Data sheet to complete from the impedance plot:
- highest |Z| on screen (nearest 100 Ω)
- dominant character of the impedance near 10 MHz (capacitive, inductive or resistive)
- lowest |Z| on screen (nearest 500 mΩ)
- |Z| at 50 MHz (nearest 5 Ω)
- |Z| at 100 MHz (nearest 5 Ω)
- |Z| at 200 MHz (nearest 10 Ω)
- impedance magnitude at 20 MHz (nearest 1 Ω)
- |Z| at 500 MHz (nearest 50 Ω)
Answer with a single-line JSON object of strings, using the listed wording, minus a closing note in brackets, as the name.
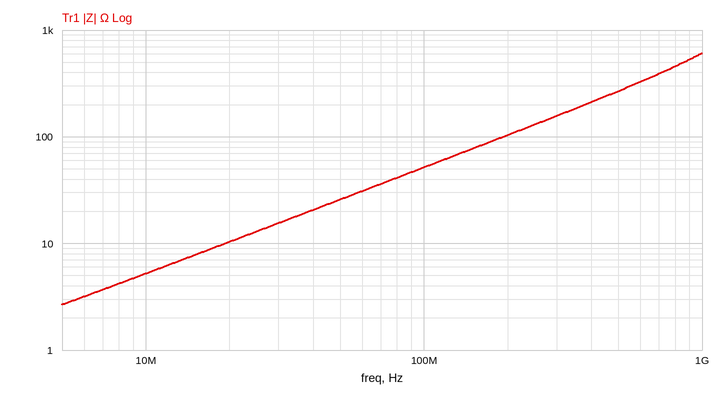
{"highest |Z| on screen": "600 Ω", "dominant character of the impedance near 10 MHz": "inductive", "lowest |Z| on screen": "2.5 Ω", "|Z| at 50 MHz": "25 Ω", "|Z| at 100 MHz": "50 Ω", "|Z| at 200 MHz": "100 Ω", "impedance magnitude at 20 MHz": "10 Ω", "|Z| at 500 MHz": "250 Ω"}
